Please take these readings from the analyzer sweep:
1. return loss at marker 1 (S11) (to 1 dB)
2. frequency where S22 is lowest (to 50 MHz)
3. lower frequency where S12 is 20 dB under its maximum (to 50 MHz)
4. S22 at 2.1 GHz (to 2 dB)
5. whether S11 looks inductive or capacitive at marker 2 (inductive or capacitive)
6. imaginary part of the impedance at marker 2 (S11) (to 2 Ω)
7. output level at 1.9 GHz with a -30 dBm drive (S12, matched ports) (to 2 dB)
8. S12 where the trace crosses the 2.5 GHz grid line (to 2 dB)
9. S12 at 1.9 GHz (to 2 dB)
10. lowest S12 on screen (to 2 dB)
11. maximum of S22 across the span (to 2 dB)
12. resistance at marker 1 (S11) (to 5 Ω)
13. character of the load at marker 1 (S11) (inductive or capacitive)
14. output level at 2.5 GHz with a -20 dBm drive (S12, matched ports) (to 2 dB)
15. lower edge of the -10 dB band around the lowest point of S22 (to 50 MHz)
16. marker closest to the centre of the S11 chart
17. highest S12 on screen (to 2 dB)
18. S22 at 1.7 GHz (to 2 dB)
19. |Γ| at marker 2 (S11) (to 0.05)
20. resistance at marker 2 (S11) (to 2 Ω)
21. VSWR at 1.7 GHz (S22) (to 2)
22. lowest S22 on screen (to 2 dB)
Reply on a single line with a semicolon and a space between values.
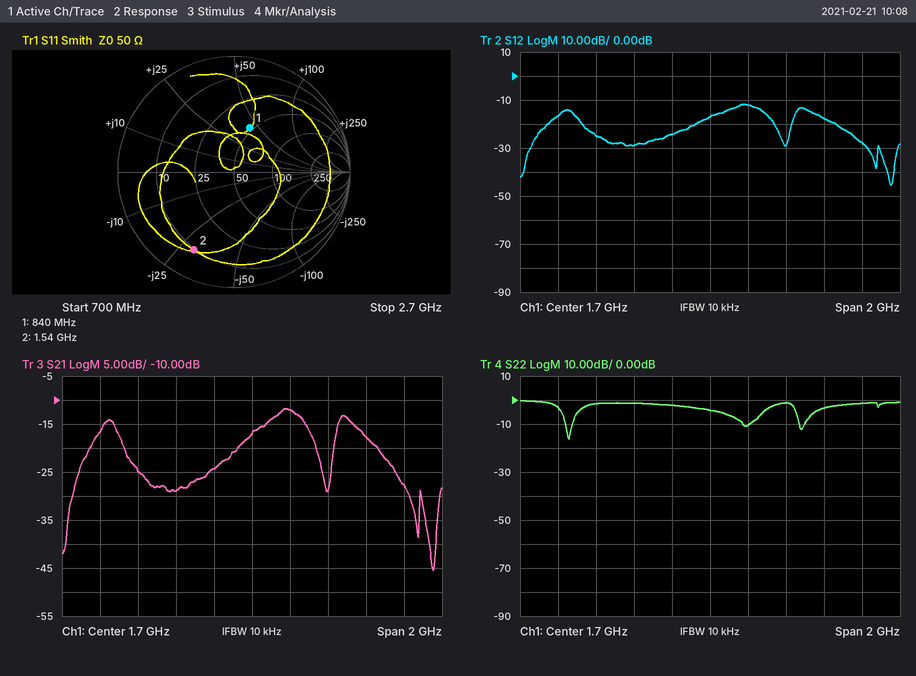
8 dB; 950 MHz; 750 MHz; -2 dB; capacitive; -30 Ω; -42 dBm; -28 dB; -12 dB; -46 dB; 0 dB; 45 Ω; inductive; -48 dBm; 950 MHz; marker 1; -12 dB; -4 dB; 0.75; 10 Ω; 4; -16 dB
